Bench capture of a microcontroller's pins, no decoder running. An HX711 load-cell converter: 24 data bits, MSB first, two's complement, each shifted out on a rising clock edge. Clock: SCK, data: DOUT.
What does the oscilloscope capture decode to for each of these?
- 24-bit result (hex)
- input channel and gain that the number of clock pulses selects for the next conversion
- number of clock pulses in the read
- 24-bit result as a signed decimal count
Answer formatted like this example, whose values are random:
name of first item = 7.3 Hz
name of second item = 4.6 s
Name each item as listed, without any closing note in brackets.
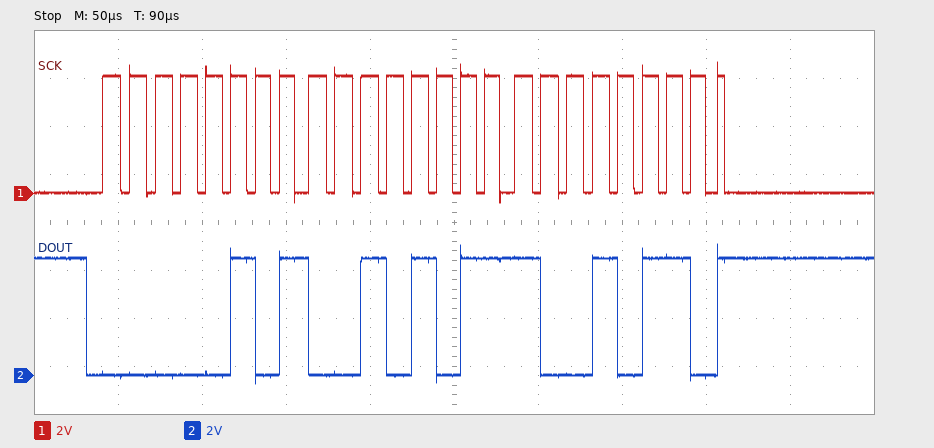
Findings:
24-bit result = 0x052B96
input channel and gain that the number of clock pulses selects for the next conversion = channel A, gain 128
number of clock pulses in the read = 25
24-bit result as a signed decimal count = 338838
